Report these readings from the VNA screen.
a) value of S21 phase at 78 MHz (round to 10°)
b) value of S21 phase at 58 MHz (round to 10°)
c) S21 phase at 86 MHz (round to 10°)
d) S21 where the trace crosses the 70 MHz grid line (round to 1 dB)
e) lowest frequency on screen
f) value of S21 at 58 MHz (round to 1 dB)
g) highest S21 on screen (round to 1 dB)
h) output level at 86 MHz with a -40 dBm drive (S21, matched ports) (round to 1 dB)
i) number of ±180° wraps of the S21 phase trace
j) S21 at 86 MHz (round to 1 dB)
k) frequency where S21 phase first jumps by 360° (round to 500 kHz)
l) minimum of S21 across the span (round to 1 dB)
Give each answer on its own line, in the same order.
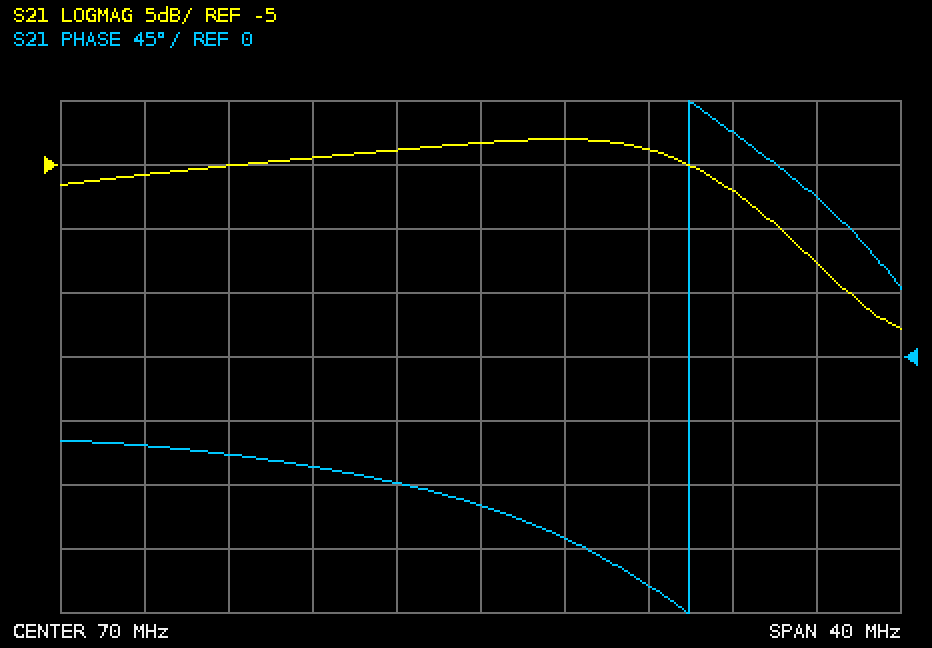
-160°
-70°
110°
-3 dB
50 MHz
-5 dB
-3 dB
-53 dBm
1
-13 dB
80.0 MHz
-18 dB
